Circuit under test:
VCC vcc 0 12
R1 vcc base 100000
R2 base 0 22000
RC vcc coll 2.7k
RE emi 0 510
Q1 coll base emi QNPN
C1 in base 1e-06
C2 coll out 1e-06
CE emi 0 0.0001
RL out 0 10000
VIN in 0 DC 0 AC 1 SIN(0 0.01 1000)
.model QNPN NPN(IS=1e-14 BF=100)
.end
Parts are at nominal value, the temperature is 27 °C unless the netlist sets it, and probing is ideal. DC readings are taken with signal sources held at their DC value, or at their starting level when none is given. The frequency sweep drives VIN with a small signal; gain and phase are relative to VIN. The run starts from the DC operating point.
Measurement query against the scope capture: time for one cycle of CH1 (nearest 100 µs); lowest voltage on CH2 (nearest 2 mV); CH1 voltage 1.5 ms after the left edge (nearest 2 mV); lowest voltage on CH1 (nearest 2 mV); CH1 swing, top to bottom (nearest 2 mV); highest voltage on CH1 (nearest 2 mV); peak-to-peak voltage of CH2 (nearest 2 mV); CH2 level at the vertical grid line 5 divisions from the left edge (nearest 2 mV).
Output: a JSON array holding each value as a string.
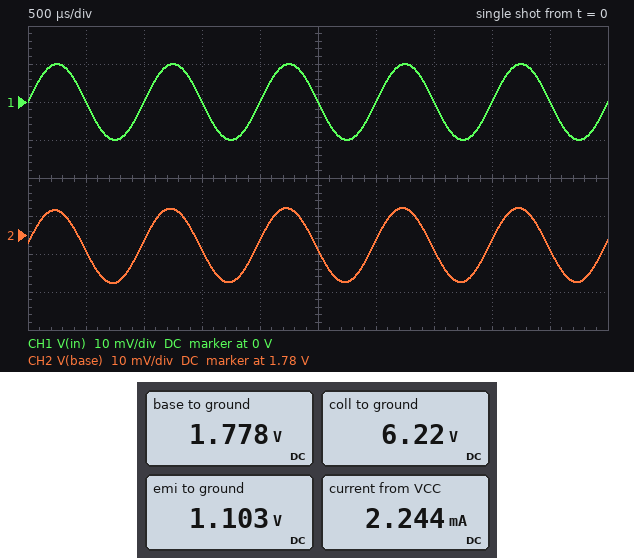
["1.0 ms", "1.768 V", "0 V", "-10 mV", "20 mV", "10 mV", "20 mV", "1.776 V"]
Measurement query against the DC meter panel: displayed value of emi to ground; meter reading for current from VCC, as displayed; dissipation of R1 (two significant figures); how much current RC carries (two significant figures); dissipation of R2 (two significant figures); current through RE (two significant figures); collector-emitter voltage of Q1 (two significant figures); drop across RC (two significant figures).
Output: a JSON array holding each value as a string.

["1.103 V", "2.244 mA", "1.0 mW", "2.1 mA", "140 µW", "2.2 mA", "5.1 V", "5.8 V"]
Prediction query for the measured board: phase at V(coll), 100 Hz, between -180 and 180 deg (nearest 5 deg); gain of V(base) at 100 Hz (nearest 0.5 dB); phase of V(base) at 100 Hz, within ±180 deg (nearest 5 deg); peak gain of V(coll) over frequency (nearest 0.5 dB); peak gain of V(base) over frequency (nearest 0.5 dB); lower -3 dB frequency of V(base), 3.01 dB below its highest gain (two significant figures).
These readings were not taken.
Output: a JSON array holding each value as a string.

["-110 deg", "-4.5 dB", "20 deg", "45.0 dB", "0 dB", "190 Hz"]
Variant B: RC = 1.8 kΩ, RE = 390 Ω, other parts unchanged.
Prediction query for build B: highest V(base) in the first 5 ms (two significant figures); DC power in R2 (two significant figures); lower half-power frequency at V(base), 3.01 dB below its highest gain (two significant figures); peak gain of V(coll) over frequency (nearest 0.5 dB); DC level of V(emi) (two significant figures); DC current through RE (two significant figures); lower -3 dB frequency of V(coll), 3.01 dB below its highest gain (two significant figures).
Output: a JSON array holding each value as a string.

["1.7 V", "130 µW", "230 Hz", "43.5 dB", "1.0 V", "2.6 mA", "330 Hz"]
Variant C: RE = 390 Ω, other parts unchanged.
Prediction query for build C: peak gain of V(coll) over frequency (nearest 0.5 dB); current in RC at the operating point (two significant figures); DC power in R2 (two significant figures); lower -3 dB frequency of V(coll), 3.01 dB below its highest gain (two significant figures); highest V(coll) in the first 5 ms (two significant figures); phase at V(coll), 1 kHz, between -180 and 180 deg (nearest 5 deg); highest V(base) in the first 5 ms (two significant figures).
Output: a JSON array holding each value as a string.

["46.5 dB", "2.6 mA", "130 µW", "330 Hz", "6.9 V", "-160 deg", "1.7 V"]
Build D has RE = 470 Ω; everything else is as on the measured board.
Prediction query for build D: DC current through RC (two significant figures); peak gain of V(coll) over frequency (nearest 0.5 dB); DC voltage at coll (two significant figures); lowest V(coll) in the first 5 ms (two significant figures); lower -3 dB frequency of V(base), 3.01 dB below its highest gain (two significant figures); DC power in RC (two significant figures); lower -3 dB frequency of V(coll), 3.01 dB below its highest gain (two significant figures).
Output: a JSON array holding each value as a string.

["2.3 mA", "45.5 dB", "5.9 V", "3.9 V", "200 Hz", "14 mW", "290 Hz"]
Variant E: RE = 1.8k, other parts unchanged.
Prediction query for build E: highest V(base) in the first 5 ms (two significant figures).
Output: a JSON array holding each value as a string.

["2.0 V"]
